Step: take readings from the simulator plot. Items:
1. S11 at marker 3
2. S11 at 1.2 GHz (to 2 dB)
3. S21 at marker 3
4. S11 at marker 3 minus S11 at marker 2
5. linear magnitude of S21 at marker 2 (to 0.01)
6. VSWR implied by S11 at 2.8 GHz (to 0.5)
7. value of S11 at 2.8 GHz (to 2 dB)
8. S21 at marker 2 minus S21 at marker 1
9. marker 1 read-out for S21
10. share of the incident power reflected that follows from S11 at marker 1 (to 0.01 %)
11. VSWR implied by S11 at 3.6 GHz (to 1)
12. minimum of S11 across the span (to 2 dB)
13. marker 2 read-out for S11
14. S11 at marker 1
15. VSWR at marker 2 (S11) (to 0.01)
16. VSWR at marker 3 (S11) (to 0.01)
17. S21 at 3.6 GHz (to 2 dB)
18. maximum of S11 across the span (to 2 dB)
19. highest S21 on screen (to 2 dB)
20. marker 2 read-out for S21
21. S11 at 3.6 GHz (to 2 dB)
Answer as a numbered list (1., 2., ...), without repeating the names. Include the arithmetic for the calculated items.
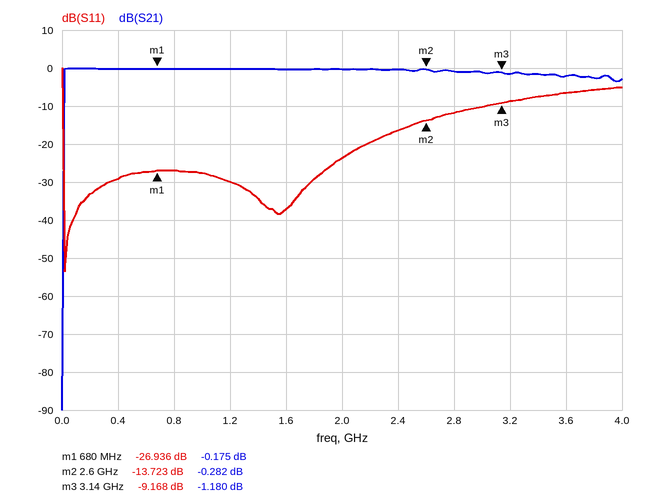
1. -9.168 dB
2. -30 dB
3. -1.180 dB
4. -9.168 − (-13.723) = 4.555 dB
5. 10^(-0.282/20) ≈ 0.97
6. |Γ| = 10^(-12/20) = 0.2512; VSWR = (1 + 0.2512)/(1 − 0.2512) ≈ 1.67, so 1.5 to the nearest 0.5
7. -12 dB
8. -0.282 − (-0.175) = -0.107 dB
9. -0.175 dB
10. 10^(-26.936/10) ≈ 0.20 %
11. |Γ| = 10^(-6/20) = 0.5012; VSWR = (1 + 0.5012)/(1 − 0.5012) ≈ 3
12. -54 dB
13. -13.723 dB
14. -26.936 dB
15. (1 + 0.2060)/(1 − 0.2060) ≈ 1.52
16. (1 + 0.3480)/(1 − 0.3480) ≈ 2.07
17. -2 dB
18. 0 dB
19. 0 dB
20. -0.282 dB
21. -6 dB
